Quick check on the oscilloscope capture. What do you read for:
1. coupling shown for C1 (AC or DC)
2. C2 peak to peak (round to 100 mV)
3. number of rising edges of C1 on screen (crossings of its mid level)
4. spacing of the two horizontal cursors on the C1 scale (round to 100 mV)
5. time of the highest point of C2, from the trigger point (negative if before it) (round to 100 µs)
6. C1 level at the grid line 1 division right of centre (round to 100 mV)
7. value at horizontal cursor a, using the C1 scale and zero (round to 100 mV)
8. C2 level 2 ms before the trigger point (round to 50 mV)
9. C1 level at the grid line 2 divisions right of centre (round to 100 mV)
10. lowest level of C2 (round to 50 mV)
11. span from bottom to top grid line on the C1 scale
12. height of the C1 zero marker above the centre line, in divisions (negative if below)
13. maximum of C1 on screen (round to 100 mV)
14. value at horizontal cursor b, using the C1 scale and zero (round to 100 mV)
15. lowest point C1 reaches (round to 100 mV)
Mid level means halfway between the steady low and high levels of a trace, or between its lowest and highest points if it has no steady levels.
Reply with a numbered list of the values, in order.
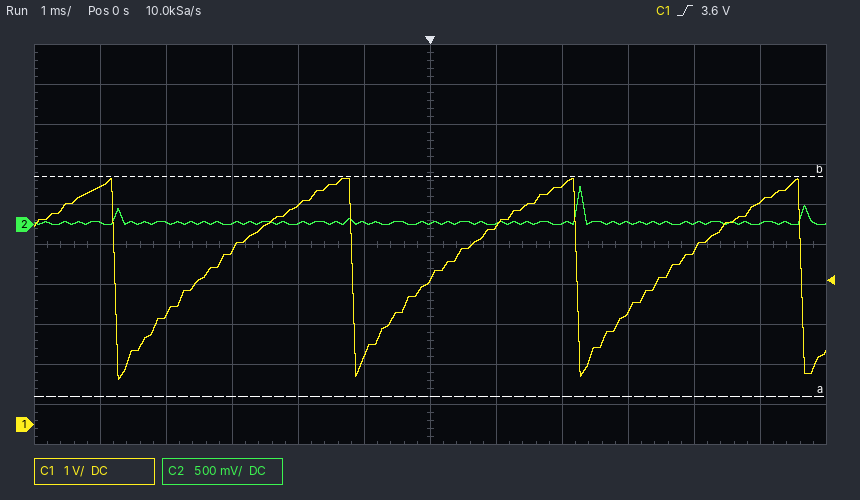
1. DC
2. 500 mV
3. 3
4. 5.5 V
5. +2.3 ms
6. 5.0 V
7. 700 mV
8. 0 mV
9. 6.0 V
10. 0 mV
11. 10 V
12. -4.5 div
13. 6.2 V
14. 6.2 V
15. 1.1 V
